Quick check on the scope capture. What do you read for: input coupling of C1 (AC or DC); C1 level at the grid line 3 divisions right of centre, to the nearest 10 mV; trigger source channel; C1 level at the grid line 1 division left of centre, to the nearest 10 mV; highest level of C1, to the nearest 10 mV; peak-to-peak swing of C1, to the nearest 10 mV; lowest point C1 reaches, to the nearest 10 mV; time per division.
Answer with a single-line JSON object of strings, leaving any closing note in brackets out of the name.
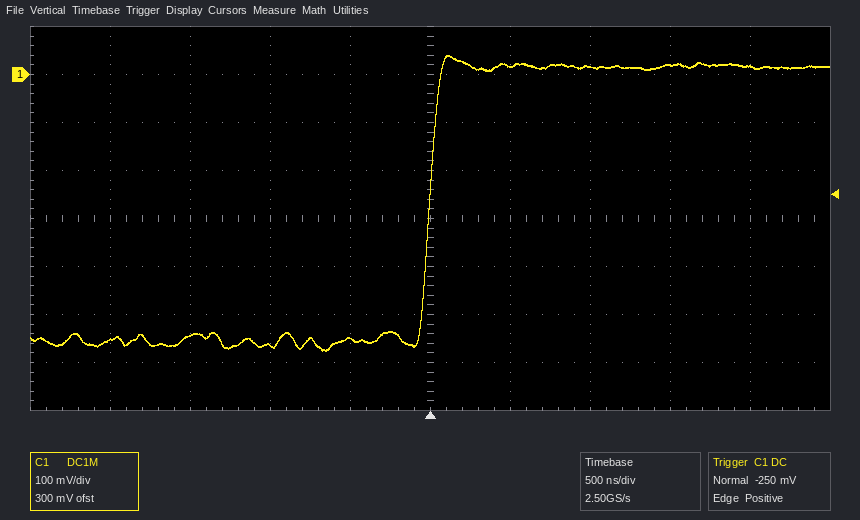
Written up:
{"input coupling of C1": "DC", "C1 level at the grid line 3 divisions right of centre, to the nearest 10 mV": "20 mV", "trigger source channel": "C1", "C1 level at the grid line 1 division left of centre, to the nearest 10 mV": "-550 mV", "highest level of C1, to the nearest 10 mV": "40 mV", "peak-to-peak swing of C1, to the nearest 10 mV": "620 mV", "lowest point C1 reaches, to the nearest 10 mV": "-580 mV", "time per division": "500 ns"}
